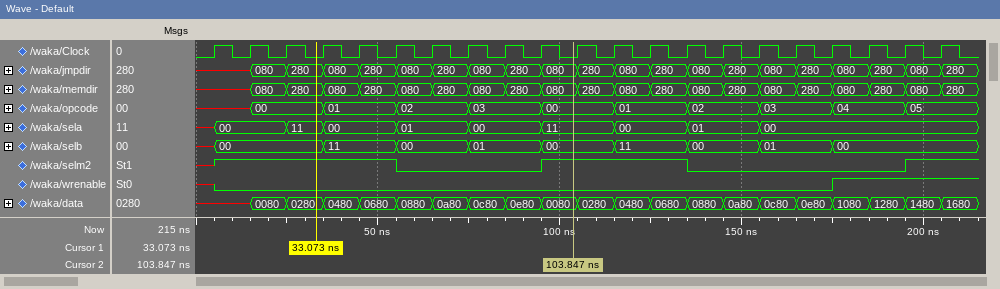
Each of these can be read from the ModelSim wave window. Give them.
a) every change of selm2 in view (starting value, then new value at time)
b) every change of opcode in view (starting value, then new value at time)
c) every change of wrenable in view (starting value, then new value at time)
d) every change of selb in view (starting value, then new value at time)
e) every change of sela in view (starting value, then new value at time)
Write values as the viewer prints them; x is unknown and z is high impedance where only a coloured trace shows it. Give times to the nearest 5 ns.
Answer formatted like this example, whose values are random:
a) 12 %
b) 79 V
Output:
a) x, 1 at 5 ns, 0 at 55 ns, 1 at 95 ns, 0 at 135 ns, 1 at 195 ns
b) x, 00 at 15 ns, 01 at 35 ns, 02 at 55 ns, 03 at 75 ns, 00 at 95 ns, 01 at 115 ns, 02 at 135 ns, 03 at 155 ns, 04 at 175 ns, 05 at 195 ns
c) x, 0 at 5 ns, 1 at 175 ns
d) x, 00 at 5 ns, 11 at 35 ns, 00 at 55 ns, 01 at 75 ns, 00 at 95 ns, 11 at 115 ns, 00 at 135 ns, 01 at 155 ns, 00 at 175 ns
e) x, 00 at 5 ns, 11 at 25 ns, 00 at 35 ns, 01 at 55 ns, 00 at 75 ns, 11 at 95 ns, 00 at 115 ns, 01 at 135 ns, 00 at 155 ns
